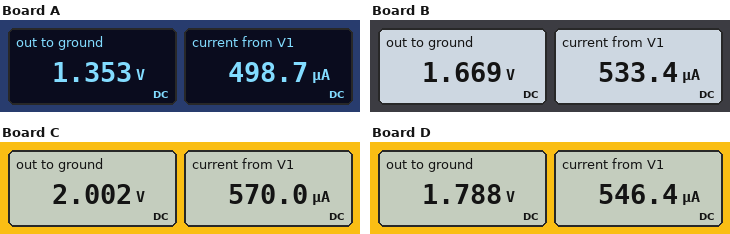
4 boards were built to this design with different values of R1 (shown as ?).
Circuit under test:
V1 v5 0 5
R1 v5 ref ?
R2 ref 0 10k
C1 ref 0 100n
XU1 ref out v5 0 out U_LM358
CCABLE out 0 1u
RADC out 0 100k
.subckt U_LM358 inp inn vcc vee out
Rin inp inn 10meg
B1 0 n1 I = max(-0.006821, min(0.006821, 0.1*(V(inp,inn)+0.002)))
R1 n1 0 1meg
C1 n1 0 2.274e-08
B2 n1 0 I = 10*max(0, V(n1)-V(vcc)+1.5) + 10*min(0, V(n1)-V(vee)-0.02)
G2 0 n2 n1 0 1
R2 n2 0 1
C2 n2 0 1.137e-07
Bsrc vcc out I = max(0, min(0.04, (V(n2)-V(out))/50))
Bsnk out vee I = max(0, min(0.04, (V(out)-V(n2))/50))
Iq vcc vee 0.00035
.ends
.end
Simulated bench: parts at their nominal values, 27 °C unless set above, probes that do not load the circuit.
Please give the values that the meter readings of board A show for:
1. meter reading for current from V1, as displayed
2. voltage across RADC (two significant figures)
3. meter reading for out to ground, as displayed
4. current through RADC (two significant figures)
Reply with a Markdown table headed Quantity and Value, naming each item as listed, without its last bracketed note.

| Quantity | Value |
|---|---|
| meter reading for current from V1, as displayed | 498.7 µA |
| voltage across RADC | 1.4 V |
| meter reading for out to ground, as displayed | 1.353 V |
| current through RADC | 14 µA |
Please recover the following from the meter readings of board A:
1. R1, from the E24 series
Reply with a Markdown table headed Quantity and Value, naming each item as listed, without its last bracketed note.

| Quantity | Value |
|---|---|
| R1, from the E24 series | 27 kΩ |
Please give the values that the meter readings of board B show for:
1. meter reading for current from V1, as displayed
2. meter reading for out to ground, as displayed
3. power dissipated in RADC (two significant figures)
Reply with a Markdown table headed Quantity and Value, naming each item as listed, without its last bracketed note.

| Quantity | Value |
|---|---|
| meter reading for current from V1, as displayed | 533.4 µA |
| meter reading for out to ground, as displayed | 1.669 V |
| power dissipated in RADC | 28 µW |
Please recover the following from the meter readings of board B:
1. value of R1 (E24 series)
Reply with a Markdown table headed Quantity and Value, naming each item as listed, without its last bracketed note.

| Quantity | Value |
|---|---|
| value of R1 | 20 kΩ |
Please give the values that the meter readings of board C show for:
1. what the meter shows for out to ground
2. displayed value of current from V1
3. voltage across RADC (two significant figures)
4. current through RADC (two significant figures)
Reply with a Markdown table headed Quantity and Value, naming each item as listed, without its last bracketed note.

| Quantity | Value |
|---|---|
| what the meter shows for out to ground | 2.002 V |
| displayed value of current from V1 | 570.0 µA |
| voltage across RADC | 2.0 V |
| current through RADC | 20 µA |
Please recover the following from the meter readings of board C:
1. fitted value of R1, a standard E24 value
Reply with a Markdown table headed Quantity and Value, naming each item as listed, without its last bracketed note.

| Quantity | Value |
|---|---|
| fitted value of R1, a standard E24 value | 15 kΩ |
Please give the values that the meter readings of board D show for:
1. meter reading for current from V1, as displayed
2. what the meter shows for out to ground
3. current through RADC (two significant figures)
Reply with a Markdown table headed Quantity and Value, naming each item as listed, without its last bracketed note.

| Quantity | Value |
|---|---|
| meter reading for current from V1, as displayed | 546.4 µA |
| what the meter shows for out to ground | 1.788 V |
| current through RADC | 18 µA |
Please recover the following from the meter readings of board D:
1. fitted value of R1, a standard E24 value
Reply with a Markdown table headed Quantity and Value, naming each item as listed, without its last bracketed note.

| Quantity | Value |
|---|---|
| fitted value of R1, a standard E24 value | 18 kΩ |
